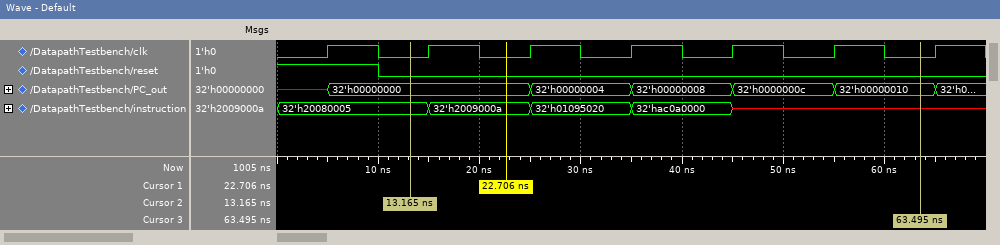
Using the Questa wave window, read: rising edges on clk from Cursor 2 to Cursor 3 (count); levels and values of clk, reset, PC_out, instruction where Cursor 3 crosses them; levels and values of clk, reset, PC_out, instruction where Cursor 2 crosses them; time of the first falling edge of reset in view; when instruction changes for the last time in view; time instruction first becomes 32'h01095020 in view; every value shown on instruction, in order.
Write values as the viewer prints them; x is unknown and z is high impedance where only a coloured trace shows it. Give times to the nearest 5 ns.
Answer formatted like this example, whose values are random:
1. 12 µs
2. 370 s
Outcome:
1. 5
2. clk=0, reset=0, PC_out=32'h00000010, instruction=x
3. clk=0, reset=0, PC_out=32'h00000000, instruction=32'h20080005
4. 10 ns
5. 45 ns
6. 25 ns
7. 32'h20080005, 32'h2009000a, 32'h01095020, 32'hac0a0000, x
